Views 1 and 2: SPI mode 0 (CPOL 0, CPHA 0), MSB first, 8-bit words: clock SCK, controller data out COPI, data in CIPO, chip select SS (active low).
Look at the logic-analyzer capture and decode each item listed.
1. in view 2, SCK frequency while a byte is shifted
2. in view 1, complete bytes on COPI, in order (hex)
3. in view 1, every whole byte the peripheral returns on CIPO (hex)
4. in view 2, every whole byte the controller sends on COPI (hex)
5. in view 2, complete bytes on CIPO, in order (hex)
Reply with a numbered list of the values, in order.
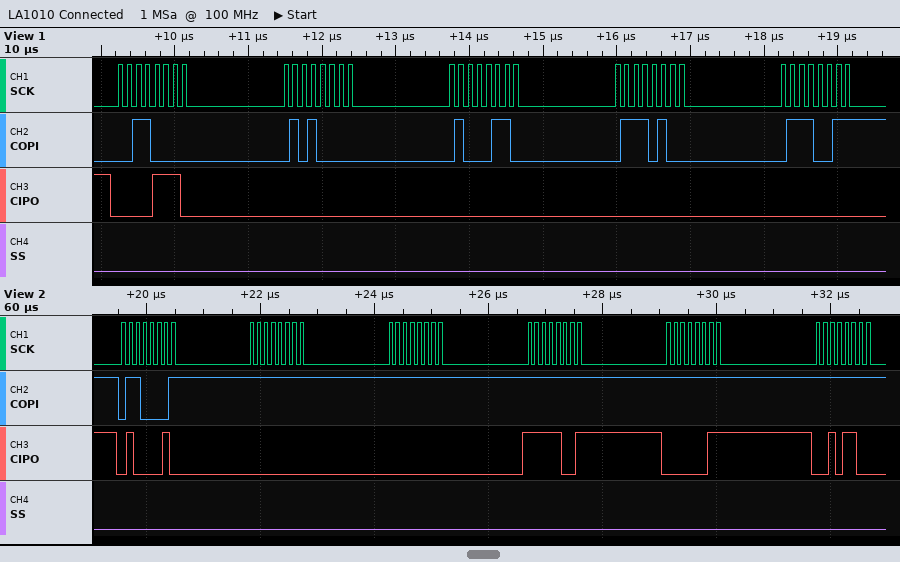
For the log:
1. 8 MHz
2. 30 50 46 74 73
3. 0E 00 00 00 00
4. 61 FF FF FF FF FF
5. 42 00 00 F9 03 2C
